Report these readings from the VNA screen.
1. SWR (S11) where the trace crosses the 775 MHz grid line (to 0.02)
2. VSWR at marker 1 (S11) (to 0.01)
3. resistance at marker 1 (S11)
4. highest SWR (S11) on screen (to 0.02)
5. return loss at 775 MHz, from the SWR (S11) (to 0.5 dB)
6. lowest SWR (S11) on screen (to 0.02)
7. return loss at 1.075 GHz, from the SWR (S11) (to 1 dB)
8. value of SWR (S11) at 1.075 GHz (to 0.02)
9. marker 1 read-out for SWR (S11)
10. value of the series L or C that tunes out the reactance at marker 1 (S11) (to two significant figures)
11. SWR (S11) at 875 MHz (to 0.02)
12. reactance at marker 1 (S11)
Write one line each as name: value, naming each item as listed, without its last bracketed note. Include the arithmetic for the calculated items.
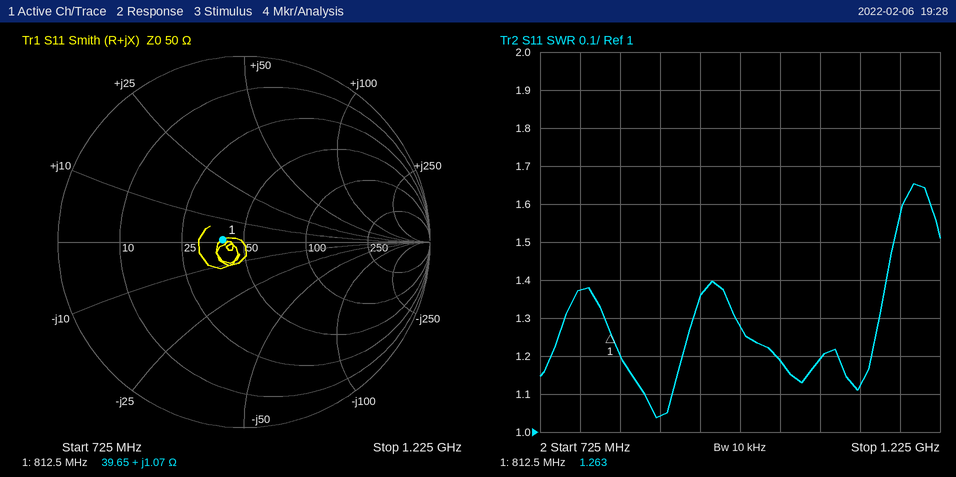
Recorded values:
SWR (S11) where the trace crosses the 775 MHz grid line: 1.38
VSWR at marker 1 (S11): 1.26
resistance at marker 1: 39.65 Ω
highest SWR (S11) on screen: 1.66
return loss at 775 MHz, from the SWR (S11): −20 log10((1.38 − 1)/(1.38 + 1)) ≈ 15.9 dB, so 16.0 dB to the nearest 0.5 dB
lowest SWR (S11) on screen: 1.04
return loss at 1.075 GHz, from the SWR (S11): −20 log10((1.2 − 1)/(1.2 + 1)) ≈ 21 dB
value of SWR (S11) at 1.075 GHz: 1.20
marker 1 read-out for SWR: 1.263
value of the series L or C that tunes out the reactance at marker 1 (S11): C = 1/(2π × 812.5 MHz × 1.07 Ω) ≈ 183 pF, so 180 pF to two significant figures
SWR (S11) at 875 MHz: 1.04
reactance at marker 1: +1.07 Ω
